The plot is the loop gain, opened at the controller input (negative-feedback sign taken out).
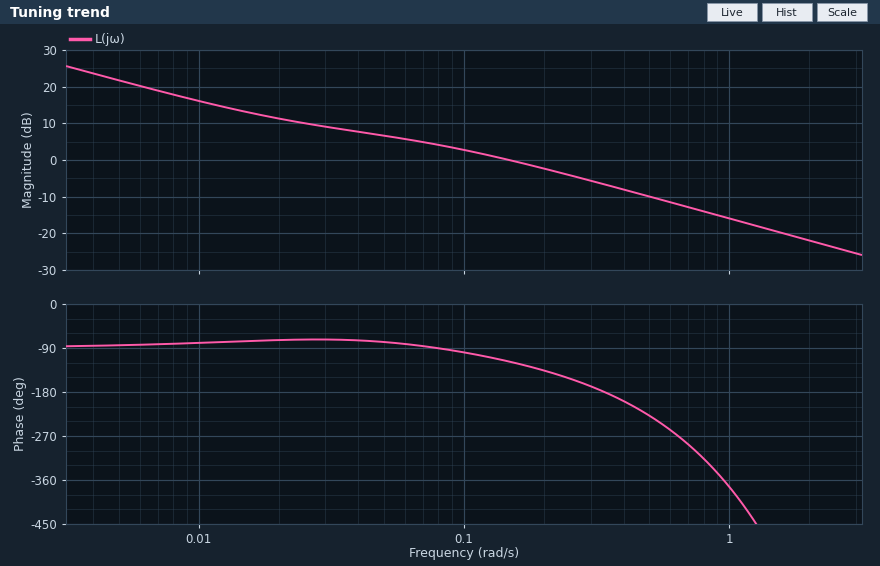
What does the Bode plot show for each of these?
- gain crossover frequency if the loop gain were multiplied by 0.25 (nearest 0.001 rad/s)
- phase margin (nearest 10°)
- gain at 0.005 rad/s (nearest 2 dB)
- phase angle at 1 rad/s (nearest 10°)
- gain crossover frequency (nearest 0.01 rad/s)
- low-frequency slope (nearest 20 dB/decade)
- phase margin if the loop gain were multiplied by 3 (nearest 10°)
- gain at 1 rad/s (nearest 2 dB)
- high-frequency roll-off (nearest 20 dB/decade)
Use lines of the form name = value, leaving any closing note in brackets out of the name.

gain crossover frequency if the loop gain were multiplied by 0.25 = 0.018 rad/s
phase margin = 60°
gain at 0.005 rad/s = 22 dB
phase angle at 1 rad/s = -370°
gain crossover frequency = 0.15 rad/s
low-frequency slope = -20 dB/decade
phase margin if the loop gain were multiplied by 3 = -40°
gain at 1 rad/s = -16 dB
high-frequency roll-off = -20 dB/decade
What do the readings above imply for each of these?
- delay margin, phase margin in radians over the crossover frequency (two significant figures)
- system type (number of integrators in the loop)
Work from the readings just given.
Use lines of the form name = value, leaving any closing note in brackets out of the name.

delay margin, phase margin in radians over the crossover frequency = 7.0 s
system type = 1
